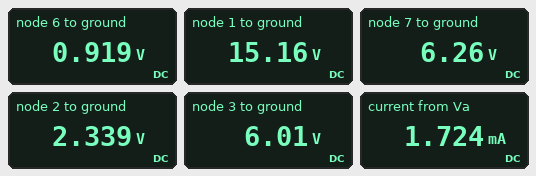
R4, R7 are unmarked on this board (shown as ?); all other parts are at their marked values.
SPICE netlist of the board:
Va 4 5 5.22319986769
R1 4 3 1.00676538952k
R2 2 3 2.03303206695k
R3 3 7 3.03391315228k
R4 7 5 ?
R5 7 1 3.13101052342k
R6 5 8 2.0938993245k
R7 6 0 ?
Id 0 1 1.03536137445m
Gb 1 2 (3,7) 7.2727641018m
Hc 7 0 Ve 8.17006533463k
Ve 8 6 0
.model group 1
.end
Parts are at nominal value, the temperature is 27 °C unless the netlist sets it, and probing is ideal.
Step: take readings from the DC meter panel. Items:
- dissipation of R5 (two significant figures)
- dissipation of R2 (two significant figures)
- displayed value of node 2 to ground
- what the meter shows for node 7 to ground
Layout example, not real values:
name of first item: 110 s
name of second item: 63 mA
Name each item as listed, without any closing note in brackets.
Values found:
dissipation of R5: 25 mW
dissipation of R2: 6.6 mW
displayed value of node 2 to ground: 2.339 V
what the meter shows for node 7 to ground: 6.26 V
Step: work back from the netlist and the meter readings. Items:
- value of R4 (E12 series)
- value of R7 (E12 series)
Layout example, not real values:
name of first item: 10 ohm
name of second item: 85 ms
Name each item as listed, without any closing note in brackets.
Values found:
value of R4: 1.5 kΩ
value of R7: 1.2 kΩ
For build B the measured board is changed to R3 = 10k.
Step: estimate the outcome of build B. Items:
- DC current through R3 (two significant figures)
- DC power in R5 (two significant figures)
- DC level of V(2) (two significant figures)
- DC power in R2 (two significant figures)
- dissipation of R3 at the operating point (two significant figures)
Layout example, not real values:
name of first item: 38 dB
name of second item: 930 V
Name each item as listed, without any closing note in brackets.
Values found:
DC current through R3: 24 µA
DC power in R5: 24 mW
DC level of V(2): 2.5 V
DC power in R2: 6.2 mW
dissipation of R3 at the operating point: 5.8 µW
